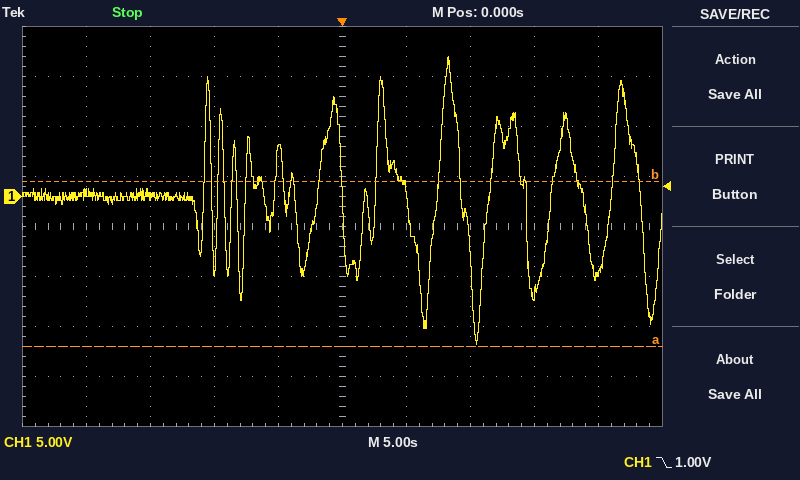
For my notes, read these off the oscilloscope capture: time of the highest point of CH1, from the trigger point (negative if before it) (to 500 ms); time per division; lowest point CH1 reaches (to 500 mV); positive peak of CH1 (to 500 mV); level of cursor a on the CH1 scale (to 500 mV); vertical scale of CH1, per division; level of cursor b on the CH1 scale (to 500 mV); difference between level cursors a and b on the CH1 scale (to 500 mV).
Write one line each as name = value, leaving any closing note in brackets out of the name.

time of the highest point of CH1, from the trigger point (negative if before it) = +8.5 s
time per division = 5 s
lowest point CH1 reaches = -15.0 V
positive peak of CH1 = 14.0 V
level of cursor a on the CH1 scale = -15.0 V
vertical scale of CH1, per division = 5 V
level of cursor b on the CH1 scale = 1.5 V
difference between level cursors a and b on the CH1 scale = 16.5 V
